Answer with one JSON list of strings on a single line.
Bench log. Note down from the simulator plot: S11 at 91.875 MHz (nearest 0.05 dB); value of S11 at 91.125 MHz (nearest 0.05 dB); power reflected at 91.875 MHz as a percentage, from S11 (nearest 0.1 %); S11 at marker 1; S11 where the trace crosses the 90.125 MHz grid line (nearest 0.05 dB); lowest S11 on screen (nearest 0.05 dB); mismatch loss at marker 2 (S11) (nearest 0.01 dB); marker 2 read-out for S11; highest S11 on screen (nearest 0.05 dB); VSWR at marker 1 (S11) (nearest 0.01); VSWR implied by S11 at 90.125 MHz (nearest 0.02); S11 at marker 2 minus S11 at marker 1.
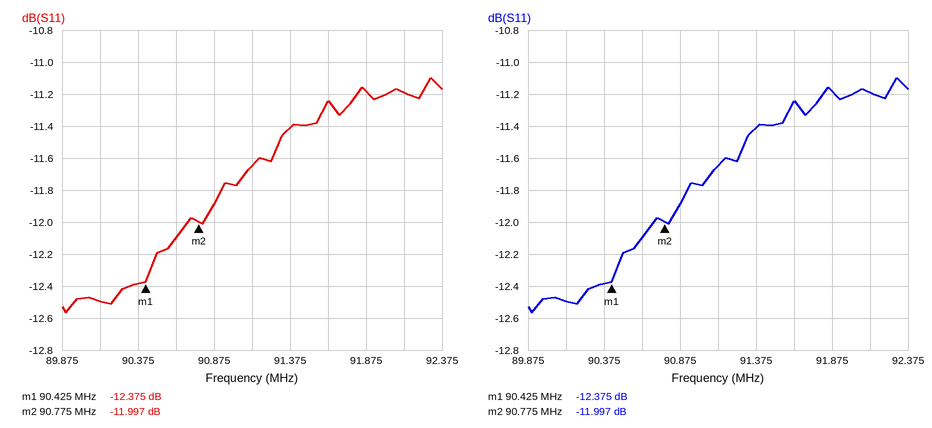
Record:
["-11.20 dB", "-11.65 dB", "7.6 %", "-12.375 dB", "-12.50 dB", "-12.55 dB", "0.28 dB", "-11.997 dB", "-11.10 dB", "1.63", "1.62", "0.378 dB"]
